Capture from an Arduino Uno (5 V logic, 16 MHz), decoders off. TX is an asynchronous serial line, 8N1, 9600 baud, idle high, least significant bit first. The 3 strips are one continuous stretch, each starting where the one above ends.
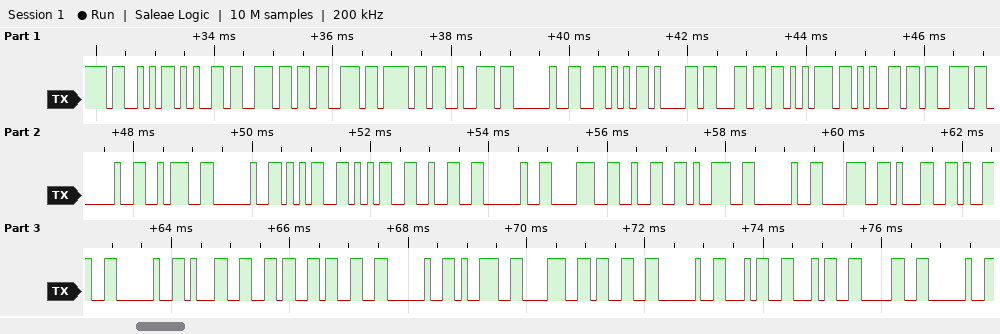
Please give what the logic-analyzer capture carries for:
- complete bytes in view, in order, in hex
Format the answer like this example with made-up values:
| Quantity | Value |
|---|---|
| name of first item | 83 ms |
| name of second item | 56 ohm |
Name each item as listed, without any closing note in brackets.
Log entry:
| Quantity | Value |
|---|---|
| complete bytes in view, in order, in hex | 53 65 6E 73 6F 72 20 56 61 6C 75 65 73 20 3A 20 35 35 32 20 38 32 39 20 38 31 39 20 31 36 33 20 39 38 33 20 34 34 30 20 |
